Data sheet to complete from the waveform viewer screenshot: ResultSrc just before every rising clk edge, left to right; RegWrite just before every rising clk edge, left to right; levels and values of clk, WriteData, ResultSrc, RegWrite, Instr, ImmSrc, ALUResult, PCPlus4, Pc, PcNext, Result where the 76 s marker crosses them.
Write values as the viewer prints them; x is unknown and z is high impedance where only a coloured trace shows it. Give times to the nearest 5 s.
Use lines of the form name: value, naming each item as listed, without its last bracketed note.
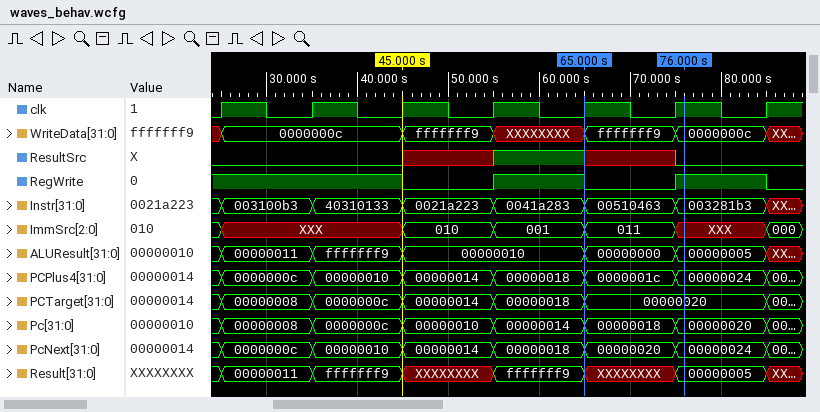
ResultSrc just before every rising clk edge, left to right: 0 0 0 x 1 x 0
RegWrite just before every rising clk edge, left to right: 1 1 1 0 1 0 1
levels and values of clk, WriteData, ResultSrc, RegWrite, Instr, ImmSrc, ALUResult, PCPlus4, Pc, PcNext, Result where the 76 s marker crosses them: clk=1, WriteData=0000000c, ResultSrc=0, RegWrite=1, Instr=003281b3, ImmSrc=XXX, ALUResult=00000005, PCPlus4=00000024, Pc=00000020, PcNext=00000024, Result=00000005
